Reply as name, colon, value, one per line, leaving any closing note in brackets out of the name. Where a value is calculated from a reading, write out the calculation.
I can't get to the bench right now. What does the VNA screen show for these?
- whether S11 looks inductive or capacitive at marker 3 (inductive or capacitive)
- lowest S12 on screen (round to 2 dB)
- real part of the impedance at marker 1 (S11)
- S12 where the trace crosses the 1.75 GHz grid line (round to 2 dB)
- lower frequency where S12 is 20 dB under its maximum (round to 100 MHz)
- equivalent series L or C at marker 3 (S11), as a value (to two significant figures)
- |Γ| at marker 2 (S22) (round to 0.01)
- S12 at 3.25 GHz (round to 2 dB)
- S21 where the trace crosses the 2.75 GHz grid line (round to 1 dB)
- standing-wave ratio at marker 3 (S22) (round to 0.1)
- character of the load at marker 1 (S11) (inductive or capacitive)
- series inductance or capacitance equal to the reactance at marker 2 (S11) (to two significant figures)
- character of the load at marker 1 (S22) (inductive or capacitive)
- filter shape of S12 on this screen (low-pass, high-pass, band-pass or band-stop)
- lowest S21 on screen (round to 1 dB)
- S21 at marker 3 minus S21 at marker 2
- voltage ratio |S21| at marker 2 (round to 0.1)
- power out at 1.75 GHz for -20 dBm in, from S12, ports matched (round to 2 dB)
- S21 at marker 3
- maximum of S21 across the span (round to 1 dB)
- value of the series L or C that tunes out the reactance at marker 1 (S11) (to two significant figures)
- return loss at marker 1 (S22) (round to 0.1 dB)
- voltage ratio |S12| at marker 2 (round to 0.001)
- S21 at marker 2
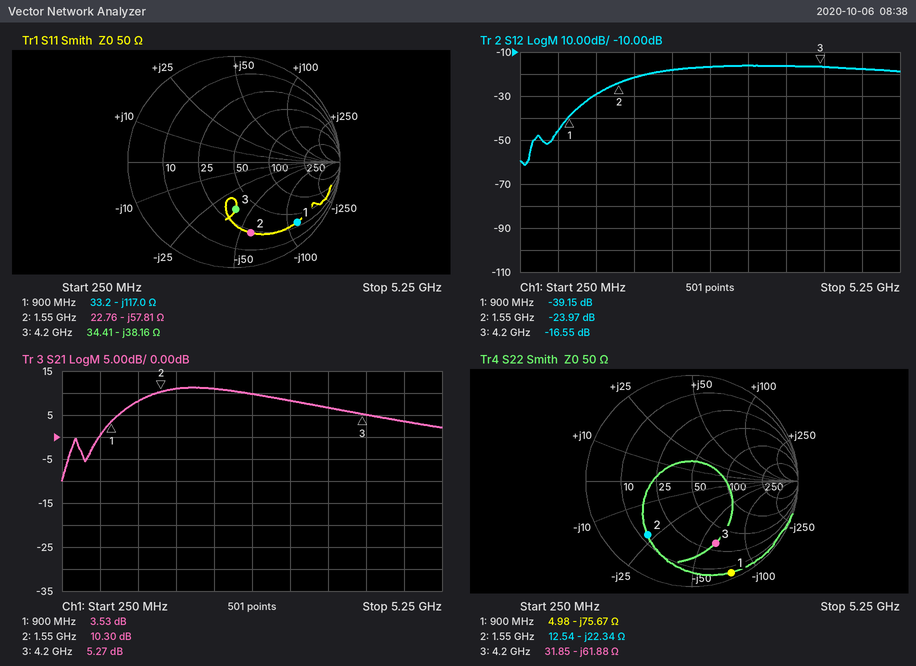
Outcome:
whether S11 looks inductive or capacitive at marker 3: capacitive
lowest S12 on screen: -62 dB
real part of the impedance at marker 1: 33.2 Ω
S12 where the trace crosses the 1.75 GHz grid line: -22 dB
lower frequency where S12 is 20 dB under its maximum: 1.0 GHz
equivalent series L or C at marker 3 (S11), as a value: C = 1/(2π × 4.2 GHz × 38.16 Ω) ≈ 993 fF, so 990 fF to two significant figures
|Γ| at marker 2 (S22): 0.66
S12 at 3.25 GHz: -16 dB
S21 where the trace crosses the 2.75 GHz grid line: 10 dB
standing-wave ratio at marker 3 (S22): 4.4
character of the load at marker 1 (S11): capacitive
series inductance or capacitance equal to the reactance at marker 2 (S11): C = 1/(2π × 1.55 GHz × 57.81 Ω) ≈ 1.8 pF
character of the load at marker 1 (S22): capacitive
filter shape of S12 on this screen: high-pass
lowest S21 on screen: -10 dB
S21 at marker 3 minus S21 at marker 2: 5.27 − (10.3) = -5.03 dB
voltage ratio |S21| at marker 2: 10^(10.3/20) ≈ 3.3
power out at 1.75 GHz for -20 dBm in, from S12, ports matched: -20 dBm + (-22 dB) = -42 dBm
S21 at marker 3: 5.27 dB
maximum of S21 across the span: 11 dB
value of the series L or C that tunes out the reactance at marker 1 (S11): L = 117 Ω/(2π × 900 MHz) ≈ 21 nH
return loss at marker 1 (S22): 0.5 dB
voltage ratio |S12| at marker 2: 10^(-23.97/20) ≈ 0.063
S21 at marker 2: 10.30 dB
